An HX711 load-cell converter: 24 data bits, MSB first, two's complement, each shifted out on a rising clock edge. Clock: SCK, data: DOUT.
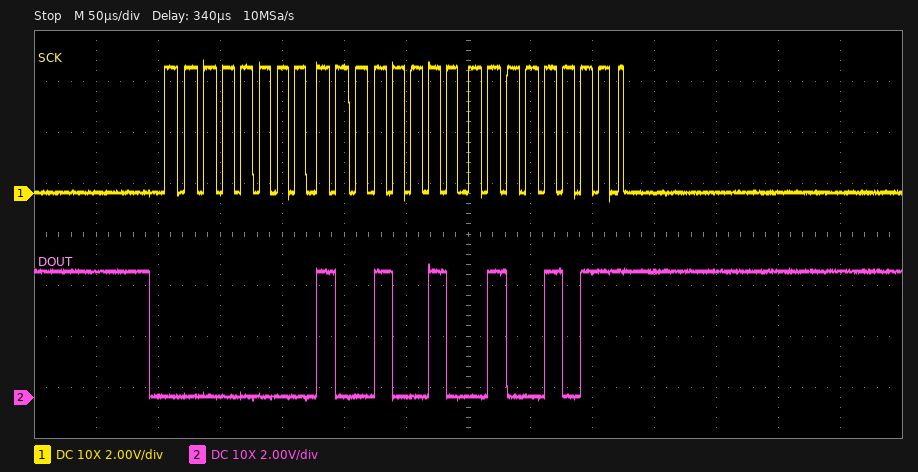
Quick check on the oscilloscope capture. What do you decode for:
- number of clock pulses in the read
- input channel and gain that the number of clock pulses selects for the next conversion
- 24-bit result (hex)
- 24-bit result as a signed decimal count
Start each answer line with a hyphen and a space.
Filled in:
- 25
- channel A, gain 128
- 0x00924B
- 37451
